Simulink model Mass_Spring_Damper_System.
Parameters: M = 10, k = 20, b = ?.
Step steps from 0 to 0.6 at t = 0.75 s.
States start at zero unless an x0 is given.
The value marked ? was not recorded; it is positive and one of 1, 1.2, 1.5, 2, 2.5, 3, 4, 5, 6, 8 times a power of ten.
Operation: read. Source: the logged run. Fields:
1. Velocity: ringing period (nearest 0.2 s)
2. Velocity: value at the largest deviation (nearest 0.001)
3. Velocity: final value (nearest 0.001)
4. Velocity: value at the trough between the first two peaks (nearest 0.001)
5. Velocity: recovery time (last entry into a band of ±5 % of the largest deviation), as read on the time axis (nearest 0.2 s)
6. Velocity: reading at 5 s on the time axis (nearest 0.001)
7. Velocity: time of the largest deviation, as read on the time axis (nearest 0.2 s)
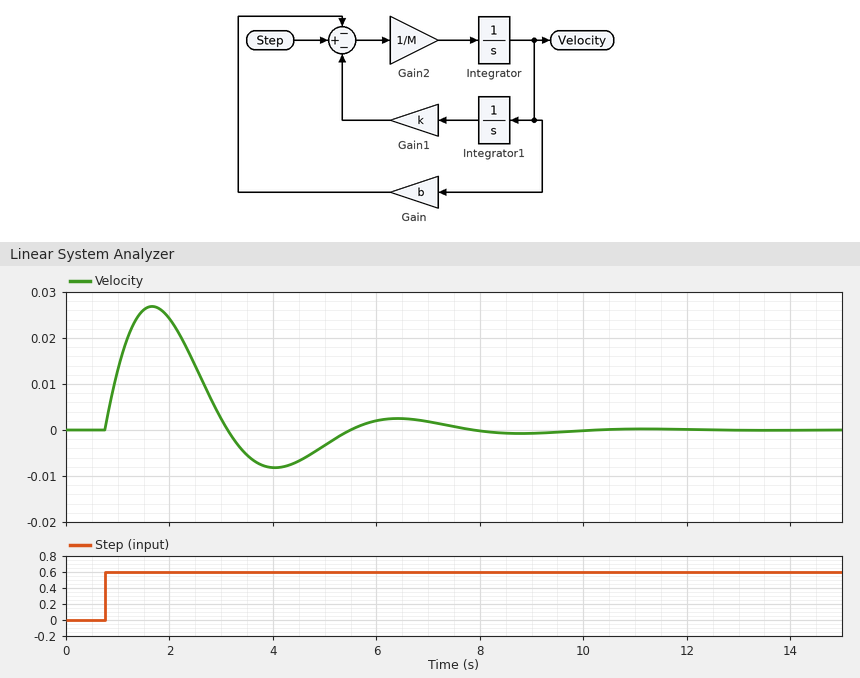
4.8 s
0.027
0.000
-0.008
7.2 s
-0.003
1.6 s
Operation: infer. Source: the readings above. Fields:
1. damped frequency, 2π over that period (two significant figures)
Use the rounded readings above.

1.3 rad/s
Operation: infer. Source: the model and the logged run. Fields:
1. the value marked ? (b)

10
